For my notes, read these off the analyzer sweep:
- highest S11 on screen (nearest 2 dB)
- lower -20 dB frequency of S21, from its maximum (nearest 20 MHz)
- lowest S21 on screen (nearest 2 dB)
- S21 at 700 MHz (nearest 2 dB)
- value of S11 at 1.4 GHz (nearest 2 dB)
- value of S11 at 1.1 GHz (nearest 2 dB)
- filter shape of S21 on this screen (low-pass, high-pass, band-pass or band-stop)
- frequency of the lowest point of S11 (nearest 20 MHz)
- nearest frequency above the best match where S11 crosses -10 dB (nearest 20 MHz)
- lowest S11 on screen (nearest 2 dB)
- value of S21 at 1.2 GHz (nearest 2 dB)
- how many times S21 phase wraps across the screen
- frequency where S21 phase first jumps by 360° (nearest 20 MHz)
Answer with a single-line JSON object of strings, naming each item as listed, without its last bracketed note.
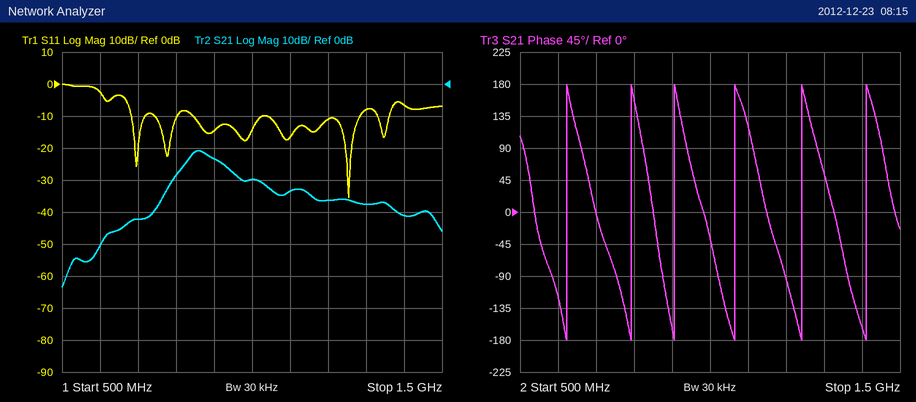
{"highest S11 on screen": "0 dB", "lower -20 dB frequency of S21, from its maximum": "740 MHz", "lowest S21 on screen": "-64 dB", "S21 at 700 MHz": "-42 dB", "value of S11 at 1.4 GHz": "-6 dB", "value of S11 at 1.1 GHz": "-16 dB", "filter shape of S21 on this screen": "band-pass", "frequency of the lowest point of S11": "1.26 GHz", "nearest frequency above the best match where S11 crosses -10 dB": "1.28 GHz", "lowest S11 on screen": "-36 dB", "value of S21 at 1.2 GHz": "-36 dB", "how many times S21 phase wraps across the screen": "6", "frequency where S21 phase first jumps by 360°": "620 MHz"}
